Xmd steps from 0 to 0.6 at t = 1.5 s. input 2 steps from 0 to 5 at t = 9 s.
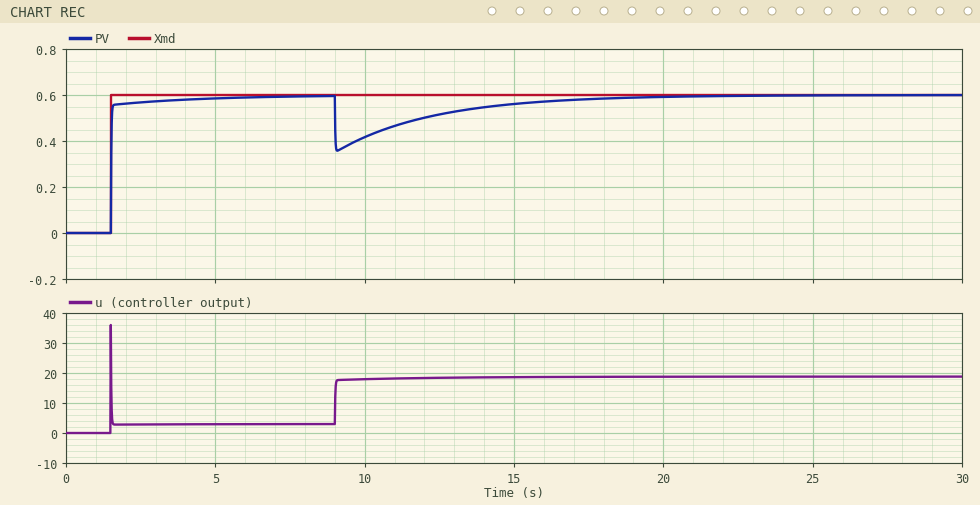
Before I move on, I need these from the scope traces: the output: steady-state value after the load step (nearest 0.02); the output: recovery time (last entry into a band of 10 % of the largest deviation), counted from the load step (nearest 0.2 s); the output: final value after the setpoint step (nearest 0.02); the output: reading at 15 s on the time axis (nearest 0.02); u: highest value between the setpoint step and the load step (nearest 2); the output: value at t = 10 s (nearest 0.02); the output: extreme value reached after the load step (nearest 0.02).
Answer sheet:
0.60
7.6 s
0.60
0.56
36
0.42
0.36
